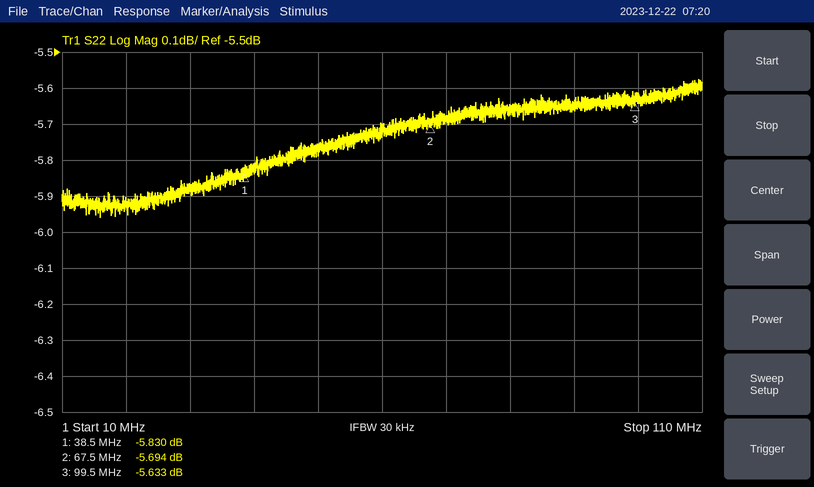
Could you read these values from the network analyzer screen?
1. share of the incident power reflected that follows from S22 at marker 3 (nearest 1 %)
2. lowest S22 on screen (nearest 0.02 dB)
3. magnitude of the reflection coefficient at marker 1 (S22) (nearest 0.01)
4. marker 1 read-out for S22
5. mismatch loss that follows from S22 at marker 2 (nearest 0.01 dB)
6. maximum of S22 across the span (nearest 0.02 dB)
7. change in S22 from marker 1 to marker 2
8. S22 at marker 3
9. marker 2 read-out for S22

27 %
-5.96 dB
0.51
-5.830 dB
1.36 dB
-5.58 dB
0.136 dB
-5.633 dB
-5.694 dB
